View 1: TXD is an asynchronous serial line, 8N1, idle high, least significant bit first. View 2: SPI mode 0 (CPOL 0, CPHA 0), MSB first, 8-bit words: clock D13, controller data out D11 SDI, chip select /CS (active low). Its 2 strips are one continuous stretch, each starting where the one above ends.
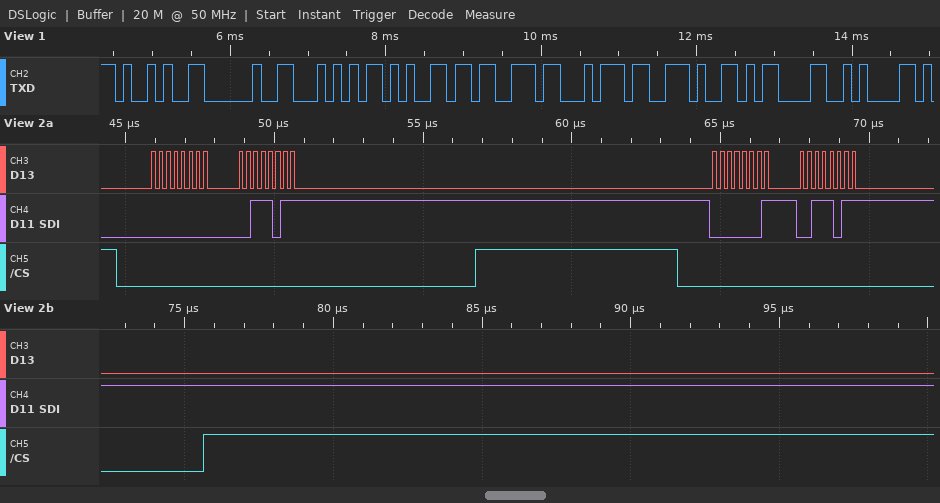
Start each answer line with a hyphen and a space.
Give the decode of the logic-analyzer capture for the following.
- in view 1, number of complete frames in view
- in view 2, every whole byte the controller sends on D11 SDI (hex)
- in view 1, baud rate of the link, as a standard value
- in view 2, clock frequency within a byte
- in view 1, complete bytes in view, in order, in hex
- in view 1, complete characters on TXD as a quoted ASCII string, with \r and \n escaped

- 9
- 0x00 0x3B 0x01 0x3B
- 9600 baud
- 4 MHz
- 29 20 54 65 73 74 2E 0D 0A
- ") Test.\r\n"
